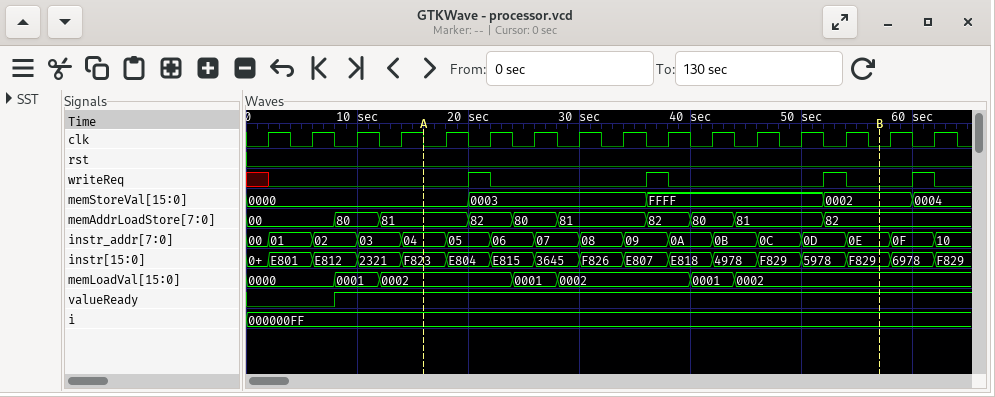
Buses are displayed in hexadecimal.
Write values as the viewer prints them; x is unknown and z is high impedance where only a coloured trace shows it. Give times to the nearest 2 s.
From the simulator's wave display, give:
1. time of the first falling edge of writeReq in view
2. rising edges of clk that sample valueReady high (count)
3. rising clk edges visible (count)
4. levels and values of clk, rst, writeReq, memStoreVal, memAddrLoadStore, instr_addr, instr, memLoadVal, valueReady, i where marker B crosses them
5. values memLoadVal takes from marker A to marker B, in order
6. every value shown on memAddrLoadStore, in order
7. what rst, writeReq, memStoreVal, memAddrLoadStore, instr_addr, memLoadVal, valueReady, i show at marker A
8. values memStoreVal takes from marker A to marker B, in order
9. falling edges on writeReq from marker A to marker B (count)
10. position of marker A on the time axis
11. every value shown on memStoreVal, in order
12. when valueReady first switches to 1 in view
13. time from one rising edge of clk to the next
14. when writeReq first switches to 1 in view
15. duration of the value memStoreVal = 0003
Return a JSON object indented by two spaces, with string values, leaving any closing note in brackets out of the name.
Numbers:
{
  "time of the first falling edge of writeReq in view": "22 s",
  "rising edges of clk that sample valueReady high": "14",
  "rising clk edges visible": "16",
  "levels and values of clk, rst, writeReq, memStoreVal, memAddrLoadStore, instr_addr, instr, memLoadVal, valueReady, i where marker B crosses them": "clk=0, rst=0, writeReq=0, memStoreVal=0002, memAddrLoadStore=82, instr_addr=0E, instr=F829, memLoadVal=0002, valueReady=1, i=000000FF",
  "values memLoadVal takes from marker A to marker B, in order": "0002, 0001, 0002, 0001, 0002",
  "every value shown on memAddrLoadStore, in order": "00, 80, 81, 82, 80, 81, 82, 80, 81, 82",
  "what rst, writeReq, memStoreVal, memAddrLoadStore, instr_addr, memLoadVal, valueReady, i show at marker A": "rst=0, writeReq=0, memStoreVal=0000, memAddrLoadStore=81, instr_addr=04, memLoadVal=0002, valueReady=1, i=000000FF",
  "values memStoreVal takes from marker A to marker B, in order": "0000, 0003, FFFF, 0002",
  "falling edges on writeReq from marker A to marker B": "3",
  "position of marker A on the time axis": "16 s",
  "every value shown on memStoreVal, in order": "0000, 0003, FFFF, 0002, 0004",
  "when valueReady first switches to 1 in view": "8 s",
  "time from one rising edge of clk to the next": "4 s",
  "when writeReq first switches to 1 in view": "20 s",
  "duration of the value memStoreVal = 0003": "16 s"
}
